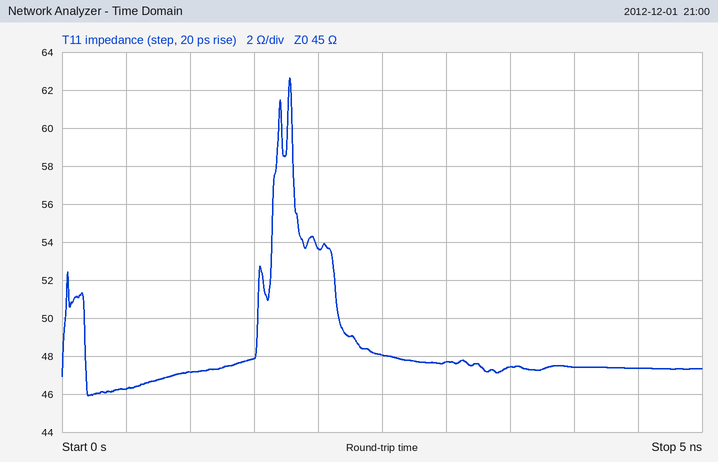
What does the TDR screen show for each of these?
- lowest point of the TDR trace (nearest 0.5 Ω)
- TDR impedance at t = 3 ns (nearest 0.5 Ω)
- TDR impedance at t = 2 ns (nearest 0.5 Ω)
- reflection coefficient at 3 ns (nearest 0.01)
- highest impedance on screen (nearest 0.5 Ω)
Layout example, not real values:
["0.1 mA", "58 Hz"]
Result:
["46.0 Ω", "47.5 Ω", "53.5 Ω", "+0.03", "62.5 Ω"]
